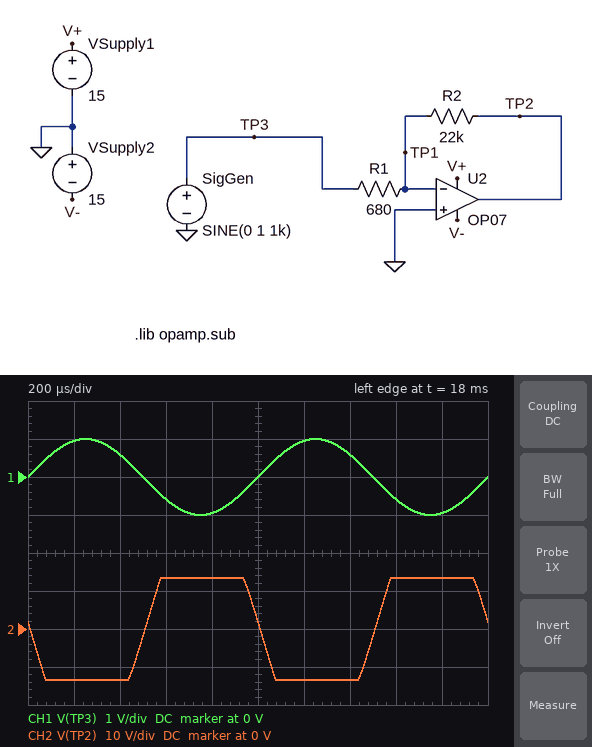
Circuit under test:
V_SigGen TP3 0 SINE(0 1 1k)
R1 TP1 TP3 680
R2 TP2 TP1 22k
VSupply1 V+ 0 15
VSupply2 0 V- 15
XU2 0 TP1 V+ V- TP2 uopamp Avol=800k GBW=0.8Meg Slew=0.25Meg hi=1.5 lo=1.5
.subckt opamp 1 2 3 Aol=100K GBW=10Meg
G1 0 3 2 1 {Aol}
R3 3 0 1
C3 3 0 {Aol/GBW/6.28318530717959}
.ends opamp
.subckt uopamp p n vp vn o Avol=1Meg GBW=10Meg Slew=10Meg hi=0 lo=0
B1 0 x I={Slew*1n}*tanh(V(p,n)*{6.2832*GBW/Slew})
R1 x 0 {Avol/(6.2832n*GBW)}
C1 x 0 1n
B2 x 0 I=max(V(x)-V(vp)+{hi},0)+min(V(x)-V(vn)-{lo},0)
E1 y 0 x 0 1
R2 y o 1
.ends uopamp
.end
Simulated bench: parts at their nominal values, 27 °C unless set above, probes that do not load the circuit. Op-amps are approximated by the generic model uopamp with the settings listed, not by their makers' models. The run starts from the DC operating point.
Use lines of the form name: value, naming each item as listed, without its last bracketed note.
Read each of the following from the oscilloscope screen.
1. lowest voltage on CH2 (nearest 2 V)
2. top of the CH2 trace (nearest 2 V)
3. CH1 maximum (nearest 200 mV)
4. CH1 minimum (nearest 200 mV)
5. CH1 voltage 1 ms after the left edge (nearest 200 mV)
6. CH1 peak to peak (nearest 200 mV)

lowest voltage on CH2: -14 V
top of the CH2 trace: 14 V
CH1 maximum: 1.0 V
CH1 minimum: -1.0 V
CH1 voltage 1 ms after the left edge: 0 V
CH1 peak to peak: 2.0 V
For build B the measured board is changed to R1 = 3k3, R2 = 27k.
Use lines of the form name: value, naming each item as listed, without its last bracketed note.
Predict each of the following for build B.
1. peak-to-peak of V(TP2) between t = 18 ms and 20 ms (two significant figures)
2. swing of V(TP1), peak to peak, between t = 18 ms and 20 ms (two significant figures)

peak-to-peak of V(TP2) between t = 18 ms and 20 ms: 16 V
swing of V(TP1), peak to peak, between t = 18 ms and 20 ms: 21 mV
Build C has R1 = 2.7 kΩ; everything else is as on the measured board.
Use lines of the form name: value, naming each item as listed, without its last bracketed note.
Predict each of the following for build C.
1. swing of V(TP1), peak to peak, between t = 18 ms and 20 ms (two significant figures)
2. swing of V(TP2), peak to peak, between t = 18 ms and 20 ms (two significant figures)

swing of V(TP1), peak to peak, between t = 18 ms and 20 ms: 21 mV
swing of V(TP2), peak to peak, between t = 18 ms and 20 ms: 16 V
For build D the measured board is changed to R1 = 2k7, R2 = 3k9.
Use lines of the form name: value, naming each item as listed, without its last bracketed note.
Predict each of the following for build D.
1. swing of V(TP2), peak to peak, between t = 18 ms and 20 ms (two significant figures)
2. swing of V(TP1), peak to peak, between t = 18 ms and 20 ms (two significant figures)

swing of V(TP2), peak to peak, between t = 18 ms and 20 ms: 2.9 V
swing of V(TP1), peak to peak, between t = 18 ms and 20 ms: 3.6 mV
